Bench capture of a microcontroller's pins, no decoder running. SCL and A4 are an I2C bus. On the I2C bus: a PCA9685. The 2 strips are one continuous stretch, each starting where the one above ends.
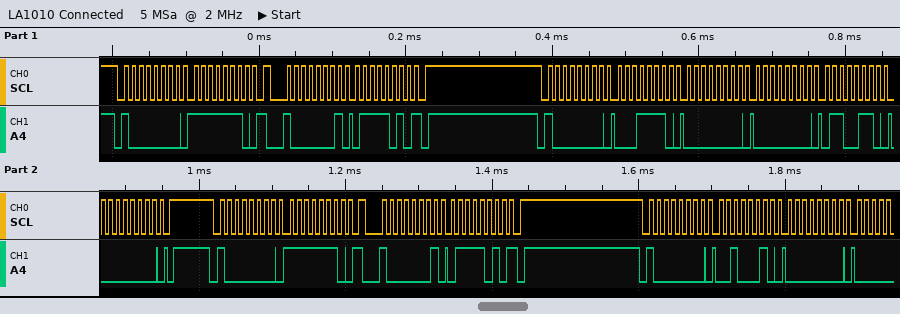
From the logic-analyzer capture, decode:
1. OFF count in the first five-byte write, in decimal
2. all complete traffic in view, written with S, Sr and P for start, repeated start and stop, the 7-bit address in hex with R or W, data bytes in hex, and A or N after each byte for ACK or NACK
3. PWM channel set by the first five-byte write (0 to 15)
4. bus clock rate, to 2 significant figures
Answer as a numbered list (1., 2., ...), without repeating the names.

1. 102
2. S 40W A FE A Sr 40R A 7A N P S 40W A 1E A 00 A 00 A 66 A 00 A P S 40W A FE A Sr 40R A 7A N P S 40W A 22 A 00 A
3. 6
4. 100 kHz
